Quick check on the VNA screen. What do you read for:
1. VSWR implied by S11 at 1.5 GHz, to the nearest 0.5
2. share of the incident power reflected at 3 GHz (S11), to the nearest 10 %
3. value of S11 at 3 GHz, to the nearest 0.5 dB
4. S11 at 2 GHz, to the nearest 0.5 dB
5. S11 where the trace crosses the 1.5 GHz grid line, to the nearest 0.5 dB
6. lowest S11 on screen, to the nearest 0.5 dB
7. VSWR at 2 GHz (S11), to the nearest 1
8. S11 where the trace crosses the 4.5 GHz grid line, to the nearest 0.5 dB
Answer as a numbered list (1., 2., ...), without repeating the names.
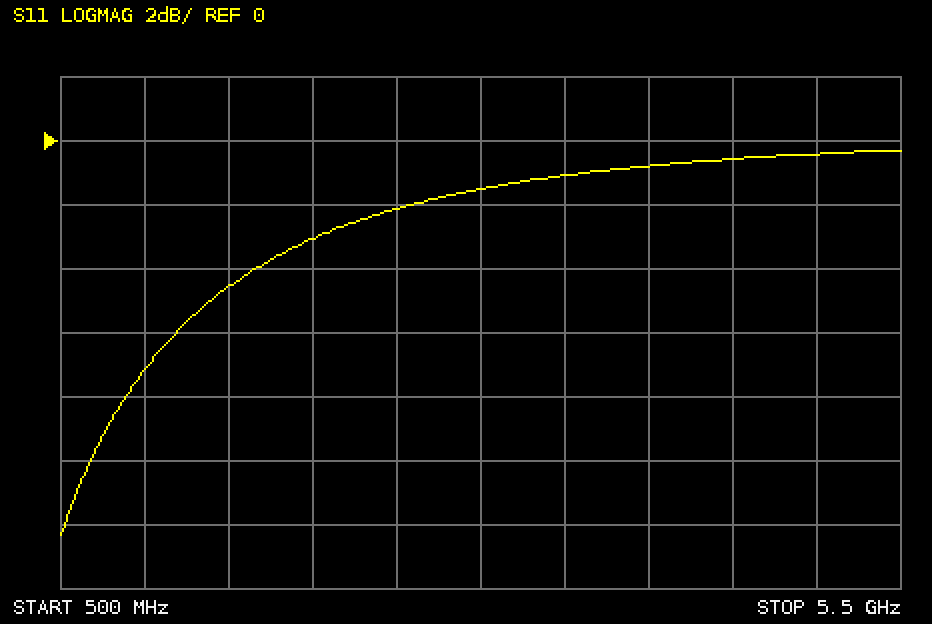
1. 4.0
2. 70 %
3. -1.5 dB
4. -3.0 dB
5. -4.5 dB
6. -12.5 dB
7. 6
8. -0.5 dB
